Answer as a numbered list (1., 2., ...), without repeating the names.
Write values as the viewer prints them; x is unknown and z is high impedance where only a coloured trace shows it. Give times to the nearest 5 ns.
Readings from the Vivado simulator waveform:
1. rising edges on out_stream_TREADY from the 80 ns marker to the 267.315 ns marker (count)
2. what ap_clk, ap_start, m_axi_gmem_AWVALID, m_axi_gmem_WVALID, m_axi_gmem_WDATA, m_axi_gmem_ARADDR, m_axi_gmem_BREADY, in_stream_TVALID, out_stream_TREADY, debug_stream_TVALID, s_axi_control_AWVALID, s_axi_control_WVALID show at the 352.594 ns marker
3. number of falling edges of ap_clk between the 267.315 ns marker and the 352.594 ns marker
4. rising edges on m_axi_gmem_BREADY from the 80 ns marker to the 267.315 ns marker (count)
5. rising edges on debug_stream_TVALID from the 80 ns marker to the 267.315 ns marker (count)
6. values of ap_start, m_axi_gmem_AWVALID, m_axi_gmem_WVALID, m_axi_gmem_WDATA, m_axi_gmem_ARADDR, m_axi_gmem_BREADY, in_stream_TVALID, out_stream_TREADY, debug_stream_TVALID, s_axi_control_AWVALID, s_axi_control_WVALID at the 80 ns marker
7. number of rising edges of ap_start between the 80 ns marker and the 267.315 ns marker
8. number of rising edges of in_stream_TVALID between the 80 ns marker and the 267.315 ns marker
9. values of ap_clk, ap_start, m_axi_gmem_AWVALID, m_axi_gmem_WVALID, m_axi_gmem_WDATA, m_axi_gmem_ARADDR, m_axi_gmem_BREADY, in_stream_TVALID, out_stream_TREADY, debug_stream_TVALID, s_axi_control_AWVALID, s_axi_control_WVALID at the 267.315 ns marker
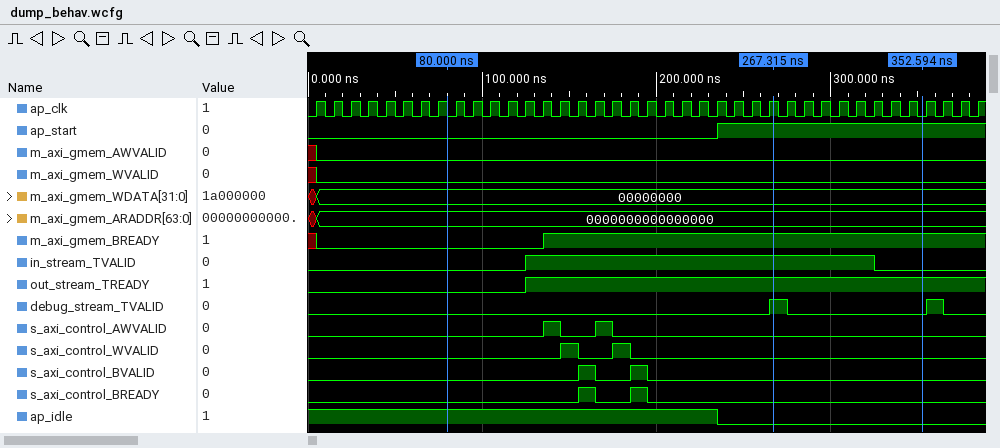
1. 1
2. ap_clk=0, ap_start=1, m_axi_gmem_AWVALID=0, m_axi_gmem_WVALID=0, m_axi_gmem_WDATA=00000000, m_axi_gmem_ARADDR=0000000000000000, m_axi_gmem_BREADY=1, in_stream_TVALID=0, out_stream_TREADY=1, debug_stream_TVALID=0, s_axi_control_AWVALID=0, s_axi_control_WVALID=0
3. 9
4. 1
5. 1
6. ap_start=0, m_axi_gmem_AWVALID=0, m_axi_gmem_WVALID=0, m_axi_gmem_WDATA=00000000, m_axi_gmem_ARADDR=0000000000000000, m_axi_gmem_BREADY=0, in_stream_TVALID=0, out_stream_TREADY=0, debug_stream_TVALID=0, s_axi_control_AWVALID=0, s_axi_control_WVALID=0
7. 1
8. 1
9. ap_clk=1, ap_start=1, m_axi_gmem_AWVALID=0, m_axi_gmem_WVALID=0, m_axi_gmem_WDATA=00000000, m_axi_gmem_ARADDR=0000000000000000, m_axi_gmem_BREADY=1, in_stream_TVALID=1, out_stream_TREADY=1, debug_stream_TVALID=1, s_axi_control_AWVALID=0, s_axi_control_WVALID=0
